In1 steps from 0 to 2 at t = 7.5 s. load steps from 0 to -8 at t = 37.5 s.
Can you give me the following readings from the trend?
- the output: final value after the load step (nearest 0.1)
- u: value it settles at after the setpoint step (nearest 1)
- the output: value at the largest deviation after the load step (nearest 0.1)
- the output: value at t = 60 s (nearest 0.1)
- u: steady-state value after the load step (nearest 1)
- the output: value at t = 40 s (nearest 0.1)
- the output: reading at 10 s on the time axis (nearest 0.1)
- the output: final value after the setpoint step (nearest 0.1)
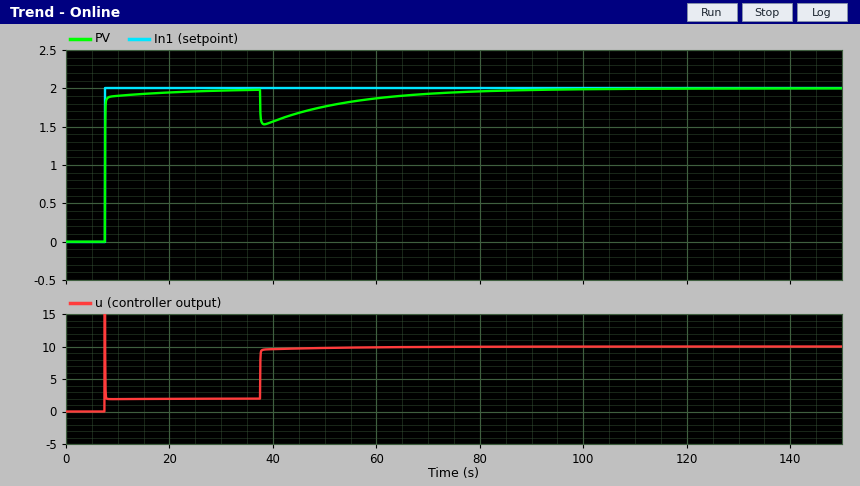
2.0
2
1.5
1.9
10
1.6
1.9
2.0
